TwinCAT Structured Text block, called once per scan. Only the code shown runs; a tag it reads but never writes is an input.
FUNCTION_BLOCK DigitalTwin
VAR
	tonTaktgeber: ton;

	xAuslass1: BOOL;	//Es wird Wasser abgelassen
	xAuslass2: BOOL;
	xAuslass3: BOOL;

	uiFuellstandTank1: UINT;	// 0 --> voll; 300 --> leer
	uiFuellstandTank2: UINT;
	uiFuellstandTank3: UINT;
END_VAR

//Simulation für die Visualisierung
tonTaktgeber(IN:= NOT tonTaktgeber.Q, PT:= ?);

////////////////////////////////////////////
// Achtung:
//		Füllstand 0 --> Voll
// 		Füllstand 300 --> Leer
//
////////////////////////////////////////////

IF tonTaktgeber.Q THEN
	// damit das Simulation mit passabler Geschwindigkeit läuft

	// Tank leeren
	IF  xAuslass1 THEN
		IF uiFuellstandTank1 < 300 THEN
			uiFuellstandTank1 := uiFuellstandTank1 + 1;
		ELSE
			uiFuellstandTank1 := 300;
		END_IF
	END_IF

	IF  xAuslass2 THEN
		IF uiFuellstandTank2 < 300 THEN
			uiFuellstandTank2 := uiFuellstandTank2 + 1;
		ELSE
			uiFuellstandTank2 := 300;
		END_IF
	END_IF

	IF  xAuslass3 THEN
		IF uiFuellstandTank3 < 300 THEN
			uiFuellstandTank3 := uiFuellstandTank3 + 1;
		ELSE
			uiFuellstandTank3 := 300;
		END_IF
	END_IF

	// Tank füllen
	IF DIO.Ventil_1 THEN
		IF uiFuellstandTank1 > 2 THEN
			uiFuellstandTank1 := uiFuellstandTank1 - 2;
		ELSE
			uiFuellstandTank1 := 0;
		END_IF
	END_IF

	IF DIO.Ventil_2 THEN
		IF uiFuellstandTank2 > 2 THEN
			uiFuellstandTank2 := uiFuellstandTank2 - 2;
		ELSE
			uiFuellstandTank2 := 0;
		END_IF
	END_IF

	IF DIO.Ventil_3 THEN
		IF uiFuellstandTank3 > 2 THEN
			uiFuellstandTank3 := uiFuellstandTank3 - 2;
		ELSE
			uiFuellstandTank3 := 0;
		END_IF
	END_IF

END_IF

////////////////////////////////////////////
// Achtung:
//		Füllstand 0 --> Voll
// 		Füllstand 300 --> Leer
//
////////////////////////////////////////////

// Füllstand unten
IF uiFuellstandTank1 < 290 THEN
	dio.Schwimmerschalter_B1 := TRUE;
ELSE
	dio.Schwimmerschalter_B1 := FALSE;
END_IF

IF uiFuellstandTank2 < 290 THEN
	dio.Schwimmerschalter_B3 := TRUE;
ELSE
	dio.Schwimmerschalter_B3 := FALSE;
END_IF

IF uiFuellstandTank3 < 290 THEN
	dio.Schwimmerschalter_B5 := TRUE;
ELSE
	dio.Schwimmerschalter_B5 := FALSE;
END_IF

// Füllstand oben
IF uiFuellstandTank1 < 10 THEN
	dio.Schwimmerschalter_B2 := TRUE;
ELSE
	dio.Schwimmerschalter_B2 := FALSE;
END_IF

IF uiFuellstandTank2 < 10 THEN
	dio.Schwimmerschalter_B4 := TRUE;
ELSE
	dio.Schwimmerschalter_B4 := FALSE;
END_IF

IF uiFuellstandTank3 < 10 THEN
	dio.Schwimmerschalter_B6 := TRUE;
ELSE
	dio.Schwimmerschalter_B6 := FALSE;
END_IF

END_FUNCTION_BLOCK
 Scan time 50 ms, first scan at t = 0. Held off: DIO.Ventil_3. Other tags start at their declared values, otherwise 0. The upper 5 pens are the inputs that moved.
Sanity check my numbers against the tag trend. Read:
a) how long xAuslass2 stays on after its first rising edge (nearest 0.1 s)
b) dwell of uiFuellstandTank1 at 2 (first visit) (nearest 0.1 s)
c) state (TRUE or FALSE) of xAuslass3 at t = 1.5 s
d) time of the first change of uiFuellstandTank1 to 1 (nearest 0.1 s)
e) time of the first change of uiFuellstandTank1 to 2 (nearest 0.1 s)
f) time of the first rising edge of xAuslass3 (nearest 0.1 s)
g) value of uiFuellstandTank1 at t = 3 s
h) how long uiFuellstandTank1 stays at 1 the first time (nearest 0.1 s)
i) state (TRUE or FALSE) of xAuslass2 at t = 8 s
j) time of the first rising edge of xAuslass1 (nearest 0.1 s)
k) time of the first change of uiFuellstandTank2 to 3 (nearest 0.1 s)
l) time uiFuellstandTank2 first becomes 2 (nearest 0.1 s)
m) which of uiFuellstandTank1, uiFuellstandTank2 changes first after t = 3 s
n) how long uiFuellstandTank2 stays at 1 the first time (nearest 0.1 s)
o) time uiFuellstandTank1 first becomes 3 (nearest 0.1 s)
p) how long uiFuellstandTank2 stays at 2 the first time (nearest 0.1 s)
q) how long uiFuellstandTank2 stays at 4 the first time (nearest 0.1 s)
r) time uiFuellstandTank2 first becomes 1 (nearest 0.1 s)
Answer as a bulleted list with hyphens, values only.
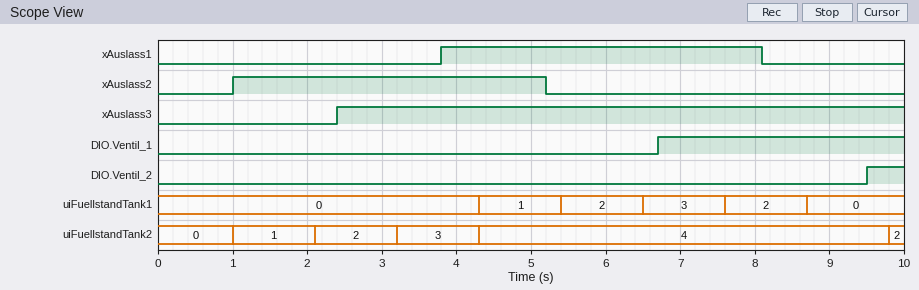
- 4.2 s
- 1.1 s
- FALSE
- 4.3 s
- 5.4 s
- 2.4 s
- 0
- 1.1 s
- FALSE
- 3.8 s
- 3.2 s
- 2.1 s
- uiFuellstandTank2
- 1.1 s
- 6.5 s
- 1.1 s
- 5.5 s
- 1.0 s
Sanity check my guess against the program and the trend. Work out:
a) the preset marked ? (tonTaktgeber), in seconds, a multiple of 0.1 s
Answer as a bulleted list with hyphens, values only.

- 1.0 s
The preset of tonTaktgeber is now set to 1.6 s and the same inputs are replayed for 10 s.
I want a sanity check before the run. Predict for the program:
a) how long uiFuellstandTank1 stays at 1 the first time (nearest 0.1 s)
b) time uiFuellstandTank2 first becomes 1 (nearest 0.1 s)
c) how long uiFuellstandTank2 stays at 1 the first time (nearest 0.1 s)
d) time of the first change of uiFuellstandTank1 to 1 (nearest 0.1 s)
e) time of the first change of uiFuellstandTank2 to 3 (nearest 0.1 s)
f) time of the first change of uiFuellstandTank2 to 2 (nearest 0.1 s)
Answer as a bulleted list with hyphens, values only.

- 1.7 s
- 1.6 s
- 1.7 s
- 5.0 s
- 5.0 s
- 3.3 s
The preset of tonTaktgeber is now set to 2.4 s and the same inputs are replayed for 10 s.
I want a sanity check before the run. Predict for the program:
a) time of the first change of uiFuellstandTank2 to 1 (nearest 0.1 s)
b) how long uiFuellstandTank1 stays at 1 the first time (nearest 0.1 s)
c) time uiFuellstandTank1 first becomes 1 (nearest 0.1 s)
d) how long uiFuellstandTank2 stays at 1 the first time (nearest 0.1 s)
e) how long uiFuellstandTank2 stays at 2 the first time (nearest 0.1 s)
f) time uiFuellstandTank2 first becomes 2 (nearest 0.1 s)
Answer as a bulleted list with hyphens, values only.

- 2.4 s
- 2.5 s
- 4.9 s
- 2.5 s
- 5.0 s
- 4.9 s
